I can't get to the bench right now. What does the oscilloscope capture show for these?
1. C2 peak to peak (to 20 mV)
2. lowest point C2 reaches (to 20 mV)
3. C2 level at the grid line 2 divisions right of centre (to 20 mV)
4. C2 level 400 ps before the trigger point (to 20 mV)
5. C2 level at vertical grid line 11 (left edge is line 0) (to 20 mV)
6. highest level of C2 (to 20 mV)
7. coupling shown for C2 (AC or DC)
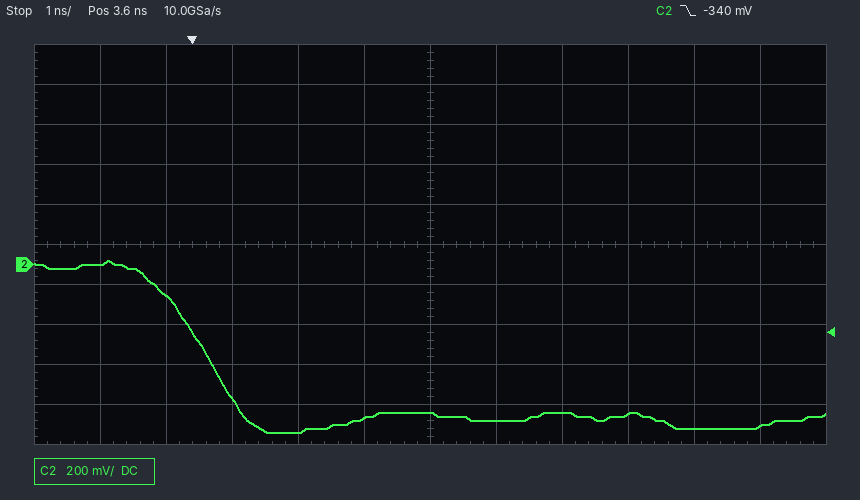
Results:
860 mV
-840 mV
-740 mV
-160 mV
-800 mV
20 mV
DC
